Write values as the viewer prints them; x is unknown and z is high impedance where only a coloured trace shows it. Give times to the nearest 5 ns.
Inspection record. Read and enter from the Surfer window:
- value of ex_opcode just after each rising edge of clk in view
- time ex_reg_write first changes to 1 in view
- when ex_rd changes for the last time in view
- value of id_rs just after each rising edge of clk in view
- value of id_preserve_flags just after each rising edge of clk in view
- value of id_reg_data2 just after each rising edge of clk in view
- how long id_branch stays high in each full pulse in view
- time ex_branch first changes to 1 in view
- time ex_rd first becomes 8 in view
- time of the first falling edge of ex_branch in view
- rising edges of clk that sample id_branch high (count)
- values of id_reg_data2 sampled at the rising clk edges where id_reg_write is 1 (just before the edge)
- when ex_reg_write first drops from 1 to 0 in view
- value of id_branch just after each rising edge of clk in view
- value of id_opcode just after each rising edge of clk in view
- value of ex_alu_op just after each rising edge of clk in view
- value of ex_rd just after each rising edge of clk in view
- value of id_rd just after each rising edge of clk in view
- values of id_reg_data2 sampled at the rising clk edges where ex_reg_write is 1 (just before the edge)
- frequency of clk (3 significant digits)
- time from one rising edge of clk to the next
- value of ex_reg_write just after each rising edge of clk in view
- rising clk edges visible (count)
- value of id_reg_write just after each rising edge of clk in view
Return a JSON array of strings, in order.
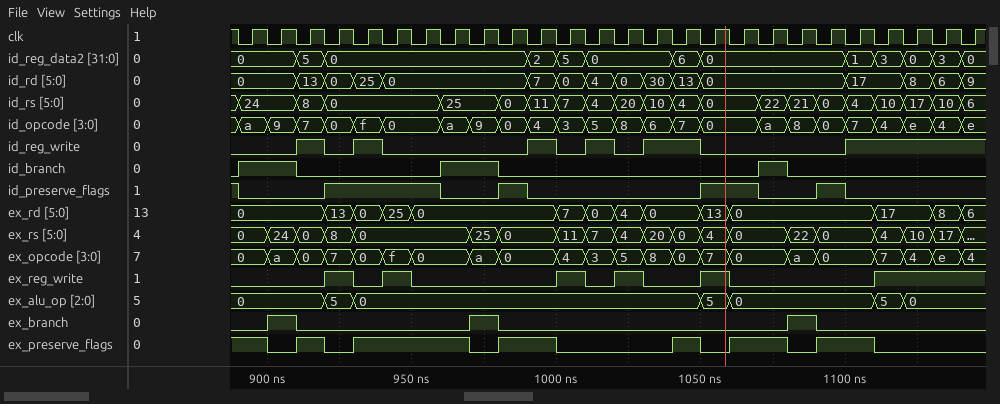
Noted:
["0, a, 0, 7, 0, f, 0, 0, a, 0, 0, 4, 3, 5, 8, 0, 7, 0, 0, a, 0, 0, 7, 4, e, 4", "920 ns", "1140 ns", "24, 24, 8, 0, 0, 0, 0, 25, 25, 0, 11, 7, 4, 20, 10, 4, 0, 0, 22, 21, 0, 4, 10, 17, 10, 6", "0 0 0 1 1 1 1 0 0 1 0 0 0 0 0 0 1 1 0 0 1 0 0 0 0 0", "0, 0, 5, 0, 0, 0, 0, 0, 0, 0, 2, 5, 0, 0, 0, 6, 0, 0, 0, 0, 0, 1, 3, 0, 3, 0", "20 ns, 20 ns, 10 ns", "900 ns", "1130 ns", "910 ns", "5", "5, 0, 2, 0, 0, 6, 1, 3, 0, 3, 0", "930 ns", "1 1 0 0 0 0 0 1 1 0 0 0 0 0 0 0 0 0 1 0 0 0 0 0 0 0", "a, 9, 7, 0, f, 0, 0, a, 9, 0, 4, 3, 5, 8, 6, 7, 0, 0, a, 8, 0, 7, 4, e, 4, e", "0, 0, 0, 5, 0, 0, 0, 0, 0, 0, 0, 0, 0, 0, 0, 0, 5, 0, 0, 0, 0, 0, 5, 0, 0, 0", "0, 0, 0, 13, 0, 25, 0, 0, 0, 0, 0, 7, 0, 4, 0, 0, 13, 0, 0, 0, 0, 0, 17, 17, 8, 6", "0, 0, 13, 0, 25, 0, 0, 0, 0, 0, 7, 0, 4, 0, 30, 13, 0, 0, 0, 0, 0, 17, 17, 8, 6, 9", "0, 0, 5, 0, 0, 3, 0, 3, 0", "100 MHz", "10 ns", "0 0 0 1 0 1 0 0 0 0 0 1 0 1 0 0 1 0 0 0 0 0 1 1 1 1", "26", "0 0 1 0 1 0 0 0 0 0 1 0 1 0 1 1 0 0 0 0 0 1 1 1 1 1"]
